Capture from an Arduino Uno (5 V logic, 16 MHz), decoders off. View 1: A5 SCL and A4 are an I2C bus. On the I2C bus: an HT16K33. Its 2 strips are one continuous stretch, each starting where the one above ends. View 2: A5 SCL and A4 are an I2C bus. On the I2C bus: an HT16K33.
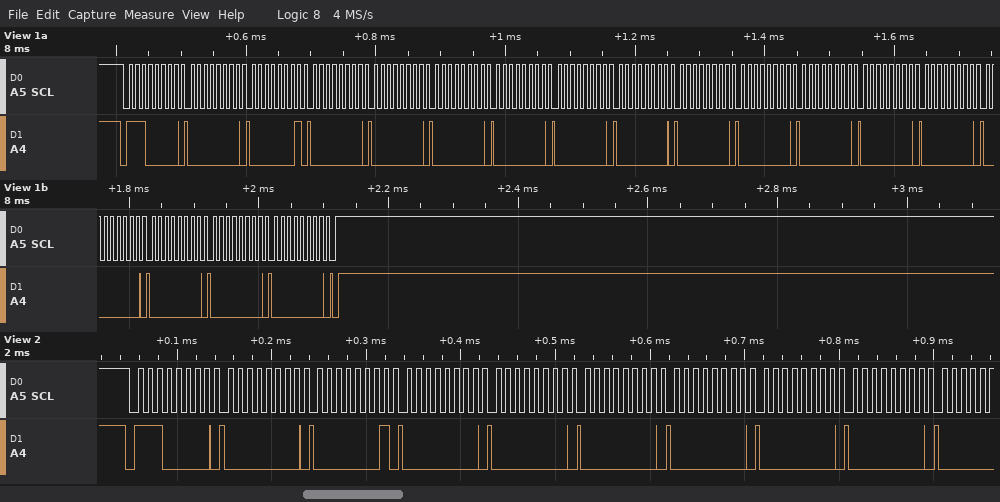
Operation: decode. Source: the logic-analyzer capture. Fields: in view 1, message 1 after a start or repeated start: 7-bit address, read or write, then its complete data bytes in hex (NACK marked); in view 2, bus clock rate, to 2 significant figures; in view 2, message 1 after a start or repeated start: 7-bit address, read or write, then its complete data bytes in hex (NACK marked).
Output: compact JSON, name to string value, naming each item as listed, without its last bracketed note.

{"in view 1, message 1 after a start or repeated start: 7-bit address, read or write, then its complete data bytes in hex": "0x70 write: 00 01 00 00 00 00 00 00 00 00 00 00 00 00 00 00 00", "in view 2, bus clock rate, to 2 significant figures": "100 kHz", "in view 2, message 1 after a start or repeated start: 7-bit address, read or write, then its complete data bytes in hex": "0x70 write: 00 01 00 00 00 00 00 00"}
